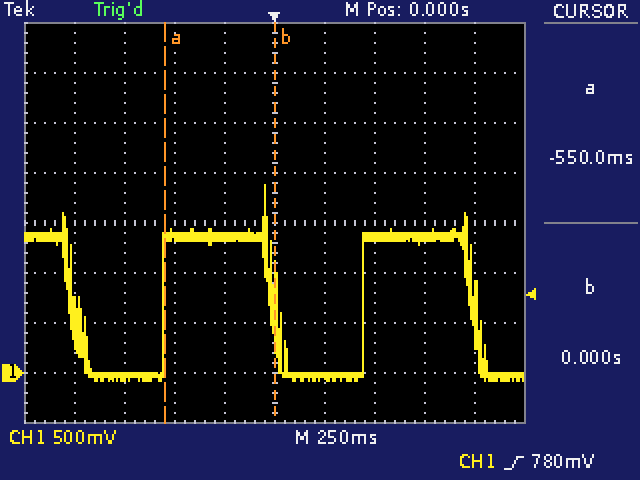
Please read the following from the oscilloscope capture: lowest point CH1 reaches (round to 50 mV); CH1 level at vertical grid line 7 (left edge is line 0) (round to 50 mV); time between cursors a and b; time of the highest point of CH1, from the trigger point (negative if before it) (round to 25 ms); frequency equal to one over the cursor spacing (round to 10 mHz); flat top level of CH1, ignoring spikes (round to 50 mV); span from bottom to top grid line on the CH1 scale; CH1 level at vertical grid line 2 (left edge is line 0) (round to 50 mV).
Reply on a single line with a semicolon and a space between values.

-100 mV; 1.35 V; 550 ms; -50 ms; 1.82 Hz; 1.35 V; 4 V; -50 mV
